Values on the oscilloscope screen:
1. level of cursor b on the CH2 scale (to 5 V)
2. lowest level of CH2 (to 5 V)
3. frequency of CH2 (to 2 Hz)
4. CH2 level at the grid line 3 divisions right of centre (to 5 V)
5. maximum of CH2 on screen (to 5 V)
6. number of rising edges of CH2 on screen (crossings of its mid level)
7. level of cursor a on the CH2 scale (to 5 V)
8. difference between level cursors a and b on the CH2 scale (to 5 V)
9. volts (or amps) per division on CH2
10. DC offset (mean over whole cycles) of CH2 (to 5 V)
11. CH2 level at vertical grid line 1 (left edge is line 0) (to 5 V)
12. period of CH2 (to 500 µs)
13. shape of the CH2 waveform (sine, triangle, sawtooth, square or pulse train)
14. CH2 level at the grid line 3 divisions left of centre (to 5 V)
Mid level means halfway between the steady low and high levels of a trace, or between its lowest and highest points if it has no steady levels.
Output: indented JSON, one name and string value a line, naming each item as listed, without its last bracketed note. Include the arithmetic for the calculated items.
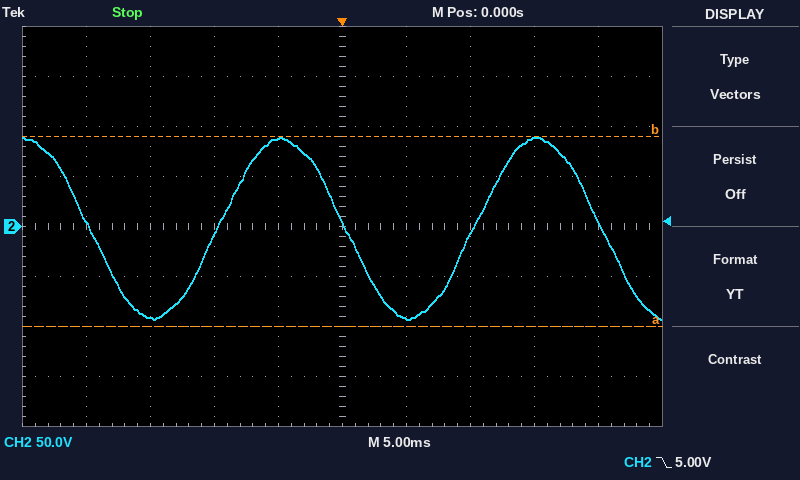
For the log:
{
  "level of cursor b on the CH2 scale": "90 V",
  "lowest level of CH2": "-95 V",
  "frequency of CH2": "1 / 20.0 ms ≈ 50 Hz",
  "CH2 level at the grid line 3 divisions right of centre": "90 V",
  "maximum of CH2 on screen": "90 V",
  "number of rising edges of CH2 on screen": "2",
  "level of cursor a on the CH2 scale": "-100 V",
  "difference between level cursors a and b on the CH2 scale": "190 V",
  "volts (or amps) per division on CH2": "50 V",
  "DC offset (mean over whole cycles) of CH2": "(90 V + (-95 V)) / 2 ≈ 0 V",
  "CH2 level at vertical grid line 1 (left edge is line 0)": "5 V",
  "period of CH2": "20.0 ms",
  "shape of the CH2 waveform": "sine",
  "CH2 level at the grid line 3 divisions left of centre": "-90 V"
}
